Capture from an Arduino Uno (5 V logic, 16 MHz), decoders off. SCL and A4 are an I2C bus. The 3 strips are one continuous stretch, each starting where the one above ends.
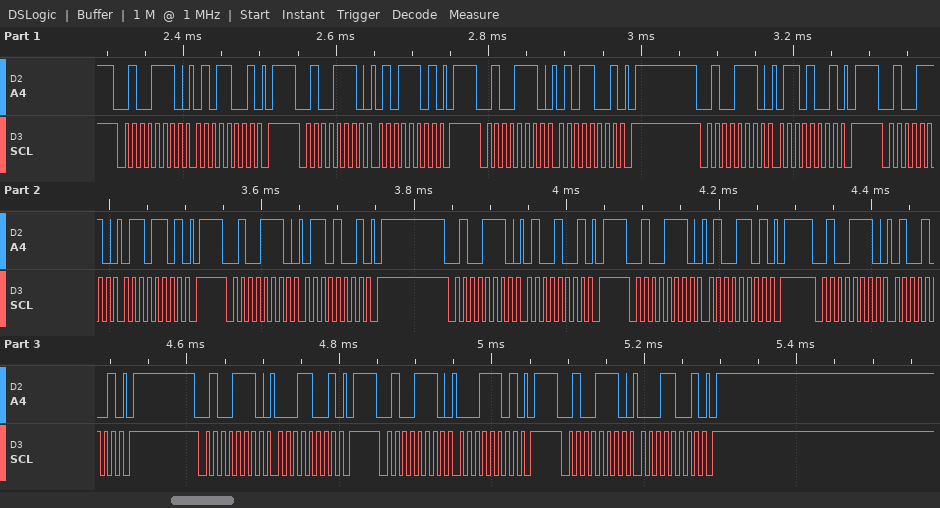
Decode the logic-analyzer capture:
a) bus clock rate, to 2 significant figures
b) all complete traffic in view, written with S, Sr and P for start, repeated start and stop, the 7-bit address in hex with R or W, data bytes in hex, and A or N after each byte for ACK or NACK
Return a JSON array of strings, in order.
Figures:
["100 kHz", "S 27W A 59 A P S 27W A 5D A P S 27W A 59 A P S 27W A 69 A P S 27W A 6D A P S 27W A 69 A P S 27W A 49 A P S 27W A 4D A P S 27W A 49 A P S 27W A 19 A P S 27W A 1D A P S 27W A 19 A P"]
